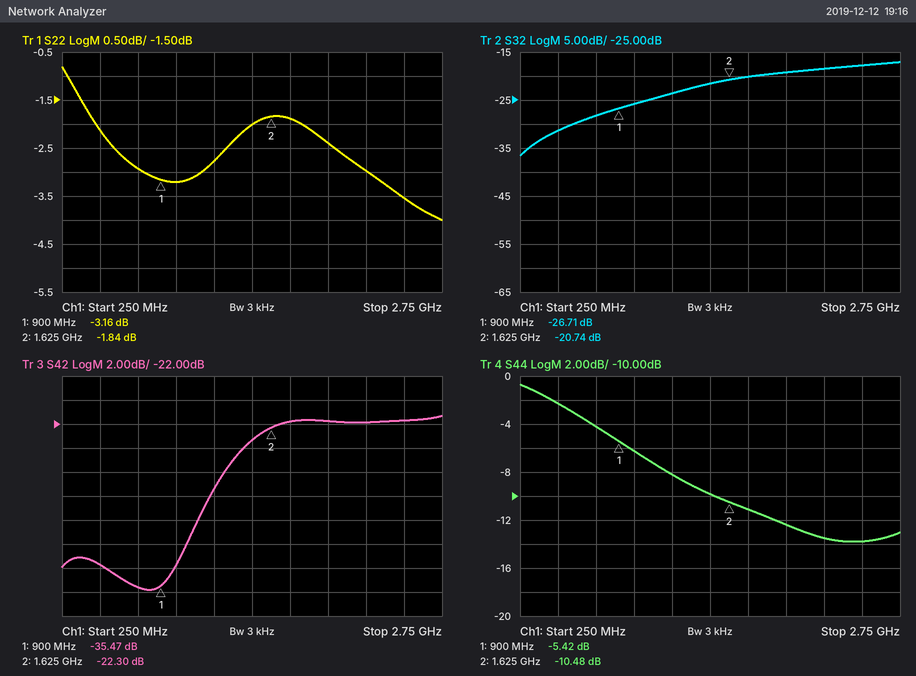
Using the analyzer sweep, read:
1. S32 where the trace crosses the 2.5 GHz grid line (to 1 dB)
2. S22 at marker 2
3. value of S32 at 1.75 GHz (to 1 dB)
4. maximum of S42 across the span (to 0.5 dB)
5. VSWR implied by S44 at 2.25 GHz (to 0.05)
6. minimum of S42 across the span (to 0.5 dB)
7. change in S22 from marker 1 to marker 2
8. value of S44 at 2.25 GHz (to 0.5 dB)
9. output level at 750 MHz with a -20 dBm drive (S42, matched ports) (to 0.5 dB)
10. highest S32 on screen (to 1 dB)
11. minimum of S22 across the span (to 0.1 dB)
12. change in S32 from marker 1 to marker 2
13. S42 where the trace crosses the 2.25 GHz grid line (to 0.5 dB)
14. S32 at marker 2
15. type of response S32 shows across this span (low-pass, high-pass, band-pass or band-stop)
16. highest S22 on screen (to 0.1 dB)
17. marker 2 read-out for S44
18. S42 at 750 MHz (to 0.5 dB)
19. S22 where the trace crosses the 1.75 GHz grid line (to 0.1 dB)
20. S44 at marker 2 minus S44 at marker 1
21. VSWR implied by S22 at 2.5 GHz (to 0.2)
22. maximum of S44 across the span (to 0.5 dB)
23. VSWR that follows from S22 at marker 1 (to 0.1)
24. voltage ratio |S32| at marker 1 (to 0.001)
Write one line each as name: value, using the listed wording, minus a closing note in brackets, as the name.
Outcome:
S32 where the trace crosses the 2.5 GHz grid line: -18 dB
S22 at marker 2: -1.84 dB
value of S32 at 1.75 GHz: -20 dB
maximum of S42 across the span: -21.5 dB
VSWR implied by S44 at 2.25 GHz: 1.55
minimum of S42 across the span: -36.0 dB
change in S22 from marker 1 to marker 2: 1.32 dB
value of S44 at 2.25 GHz: -13.5 dB
output level at 750 MHz with a -20 dBm drive (S42, matched ports): -55.5 dBm
highest S32 on screen: -17 dB
minimum of S22 across the span: -4.0 dB
change in S32 from marker 1 to marker 2: 5.97 dB
S42 where the trace crosses the 2.25 GHz grid line: -22.0 dB
S32 at marker 2: -20.74 dB
type of response S32 shows across this span: high-pass
highest S22 on screen: -0.8 dB
marker 2 read-out for S44: -10.48 dB
S42 at 750 MHz: -35.5 dB
S22 where the trace crosses the 1.75 GHz grid line: -1.9 dB
S44 at marker 2 minus S44 at marker 1: -5.06 dB
VSWR implied by S22 at 2.5 GHz: 5.0
maximum of S44 across the span: -0.5 dB
VSWR that follows from S22 at marker 1: 5.6
voltage ratio |S32| at marker 1: 0.046
